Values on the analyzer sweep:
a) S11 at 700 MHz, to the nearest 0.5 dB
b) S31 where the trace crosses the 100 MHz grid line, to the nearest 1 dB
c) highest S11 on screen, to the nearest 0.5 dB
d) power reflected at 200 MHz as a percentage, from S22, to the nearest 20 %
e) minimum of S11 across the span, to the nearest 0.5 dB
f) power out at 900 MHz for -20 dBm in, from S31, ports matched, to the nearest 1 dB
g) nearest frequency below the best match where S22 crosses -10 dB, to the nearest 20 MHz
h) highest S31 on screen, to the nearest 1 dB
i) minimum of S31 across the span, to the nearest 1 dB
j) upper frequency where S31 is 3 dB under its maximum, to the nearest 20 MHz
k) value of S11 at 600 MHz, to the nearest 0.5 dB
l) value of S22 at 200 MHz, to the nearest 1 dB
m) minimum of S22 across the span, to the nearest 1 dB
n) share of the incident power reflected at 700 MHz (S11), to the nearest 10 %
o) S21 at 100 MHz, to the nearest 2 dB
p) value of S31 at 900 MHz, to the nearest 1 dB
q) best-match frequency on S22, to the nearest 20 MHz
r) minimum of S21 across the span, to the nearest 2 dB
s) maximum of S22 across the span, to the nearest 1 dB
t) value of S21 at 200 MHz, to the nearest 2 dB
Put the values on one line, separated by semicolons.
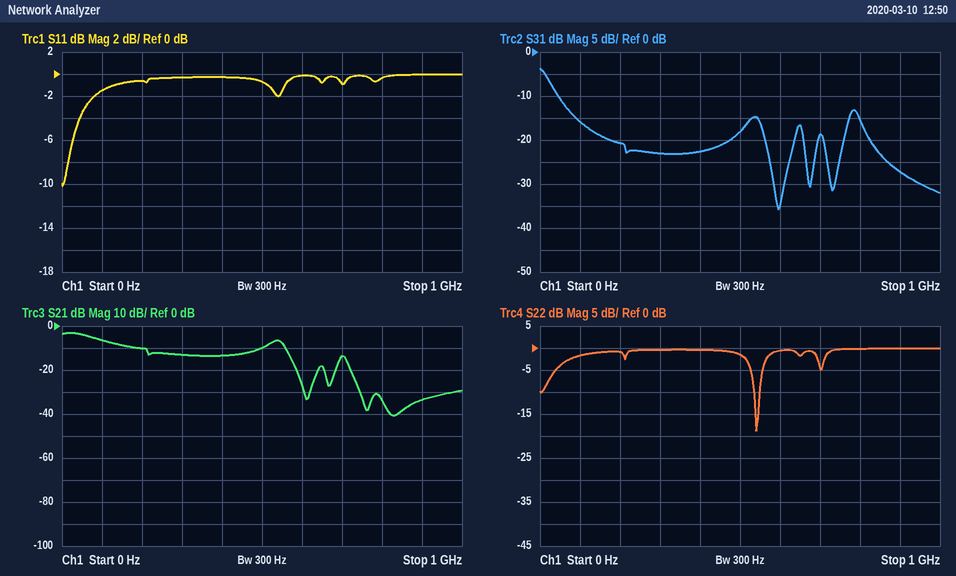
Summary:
-1.0 dB; -16 dB; 0.0 dB; 80 %; -10.0 dB; -47 dBm; 540 MHz; -4 dB; -36 dB; 20 MHz; 0.0 dB; -1 dB; -19 dB; 80 %; -6 dB; -27 dB; 540 MHz; -40 dB; 0 dB; -10 dB
